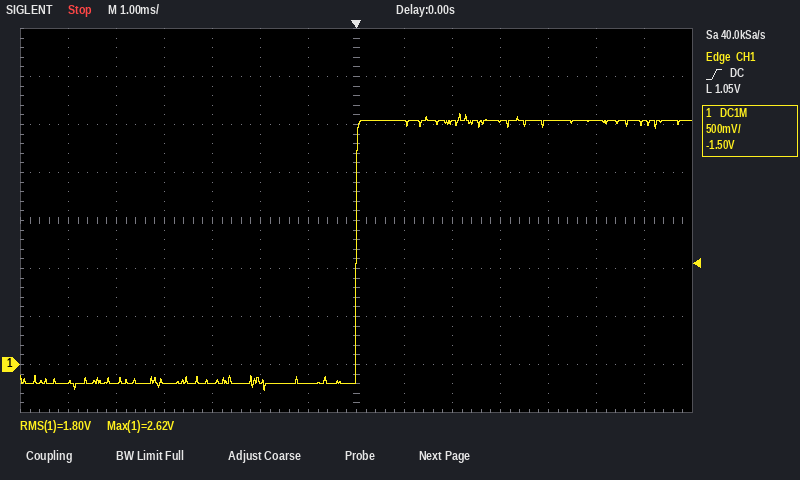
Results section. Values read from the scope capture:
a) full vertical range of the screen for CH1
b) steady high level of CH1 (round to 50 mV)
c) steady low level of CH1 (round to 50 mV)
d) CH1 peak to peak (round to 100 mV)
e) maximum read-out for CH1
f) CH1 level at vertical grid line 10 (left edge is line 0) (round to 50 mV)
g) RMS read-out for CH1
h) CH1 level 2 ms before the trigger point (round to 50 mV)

4 V
2.55 V
-200 mV
2.90 V
2.62 V
2.55 V
1.80 V
-150 mV
